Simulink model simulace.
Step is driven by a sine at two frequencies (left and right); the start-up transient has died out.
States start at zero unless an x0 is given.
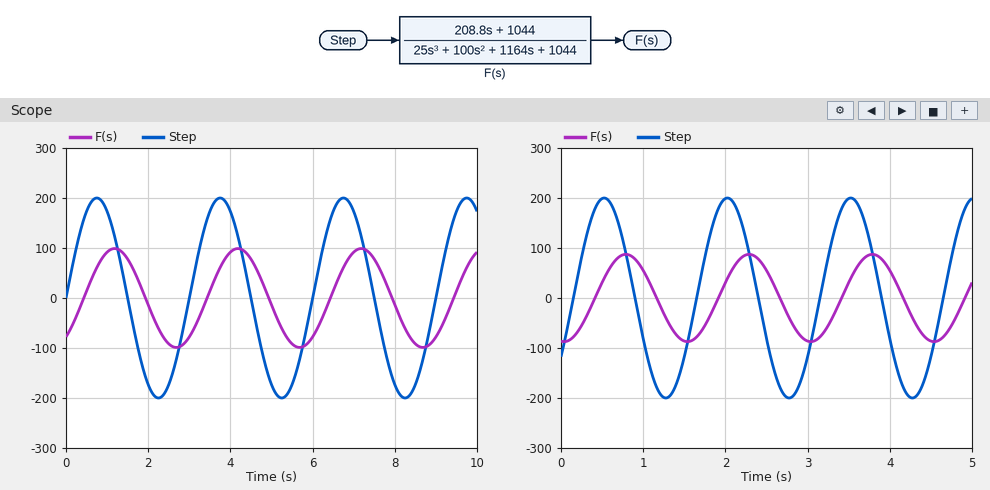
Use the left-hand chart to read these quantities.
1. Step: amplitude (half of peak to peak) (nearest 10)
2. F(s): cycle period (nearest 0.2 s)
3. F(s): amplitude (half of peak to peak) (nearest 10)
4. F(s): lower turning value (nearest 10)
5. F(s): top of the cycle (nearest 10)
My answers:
200
3.0 s
100
-100
100
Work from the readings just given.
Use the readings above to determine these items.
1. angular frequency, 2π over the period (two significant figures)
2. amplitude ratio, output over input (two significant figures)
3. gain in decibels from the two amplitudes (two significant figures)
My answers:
2.1 rad/s
0.50
-6.0 dB
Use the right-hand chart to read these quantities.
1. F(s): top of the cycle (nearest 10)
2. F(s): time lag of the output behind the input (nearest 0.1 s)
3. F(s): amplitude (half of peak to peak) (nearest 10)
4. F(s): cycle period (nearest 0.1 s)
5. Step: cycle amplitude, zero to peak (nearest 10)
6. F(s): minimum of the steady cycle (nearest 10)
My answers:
90
0.3 s
90
1.5 s
200
-90
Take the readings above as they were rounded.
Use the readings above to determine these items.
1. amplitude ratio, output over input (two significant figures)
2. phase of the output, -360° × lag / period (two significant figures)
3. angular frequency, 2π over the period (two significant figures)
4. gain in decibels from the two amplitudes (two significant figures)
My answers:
0.45
-72°
4.2 rad/s
-6.9 dB
